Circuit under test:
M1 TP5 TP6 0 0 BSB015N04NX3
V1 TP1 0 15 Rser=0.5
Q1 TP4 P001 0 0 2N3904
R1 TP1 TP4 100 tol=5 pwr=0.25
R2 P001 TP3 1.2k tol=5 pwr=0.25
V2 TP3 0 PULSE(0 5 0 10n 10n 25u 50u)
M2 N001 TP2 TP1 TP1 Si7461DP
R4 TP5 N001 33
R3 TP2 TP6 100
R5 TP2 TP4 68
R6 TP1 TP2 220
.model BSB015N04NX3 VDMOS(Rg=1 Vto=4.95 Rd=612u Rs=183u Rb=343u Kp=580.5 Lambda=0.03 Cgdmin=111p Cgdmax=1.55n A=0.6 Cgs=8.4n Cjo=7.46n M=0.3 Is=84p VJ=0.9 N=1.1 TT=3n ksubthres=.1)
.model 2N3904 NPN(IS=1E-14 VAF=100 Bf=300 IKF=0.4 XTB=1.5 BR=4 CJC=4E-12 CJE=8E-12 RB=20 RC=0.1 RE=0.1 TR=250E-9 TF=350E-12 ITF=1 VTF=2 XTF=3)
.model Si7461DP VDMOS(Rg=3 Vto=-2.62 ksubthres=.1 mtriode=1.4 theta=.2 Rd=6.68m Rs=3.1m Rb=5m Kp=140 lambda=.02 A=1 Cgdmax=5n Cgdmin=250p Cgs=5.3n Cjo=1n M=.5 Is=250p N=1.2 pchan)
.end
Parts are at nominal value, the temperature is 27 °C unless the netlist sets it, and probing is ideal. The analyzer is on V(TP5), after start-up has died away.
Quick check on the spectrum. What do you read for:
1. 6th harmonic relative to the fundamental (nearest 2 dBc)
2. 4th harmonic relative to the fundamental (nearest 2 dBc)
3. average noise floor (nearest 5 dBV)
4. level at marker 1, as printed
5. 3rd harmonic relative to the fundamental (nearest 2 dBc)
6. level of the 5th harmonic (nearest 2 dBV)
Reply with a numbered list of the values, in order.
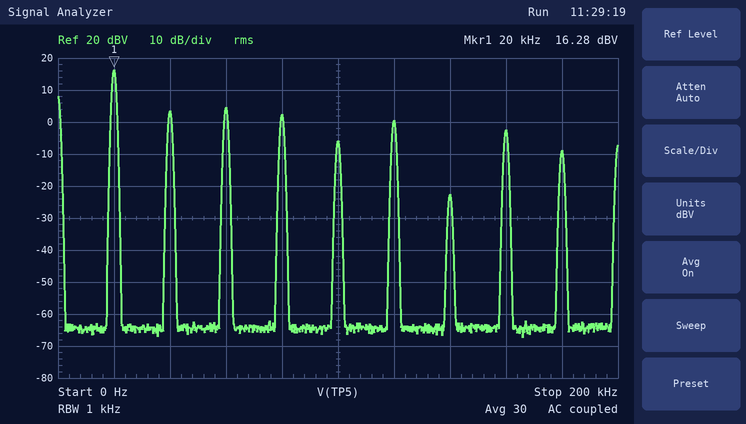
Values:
1. -16 dBc
2. -14 dBc
3. -65 dBV
4. 16.28 dBV
5. -12 dBc
6. -6 dBV
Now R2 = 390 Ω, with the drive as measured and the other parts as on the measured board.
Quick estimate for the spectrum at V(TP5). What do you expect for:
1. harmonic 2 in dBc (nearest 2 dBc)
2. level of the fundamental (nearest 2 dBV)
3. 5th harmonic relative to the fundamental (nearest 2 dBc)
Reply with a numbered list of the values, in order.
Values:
1. -14 dBc
2. 16 dBV
3. -20 dBc
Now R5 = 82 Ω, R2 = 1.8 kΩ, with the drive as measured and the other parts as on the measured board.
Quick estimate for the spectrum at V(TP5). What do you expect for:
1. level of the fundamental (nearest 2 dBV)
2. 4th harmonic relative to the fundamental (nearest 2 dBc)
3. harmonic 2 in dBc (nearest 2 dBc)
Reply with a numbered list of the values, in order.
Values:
1. 16 dBV
2. -12 dBc
3. -8 dBc
